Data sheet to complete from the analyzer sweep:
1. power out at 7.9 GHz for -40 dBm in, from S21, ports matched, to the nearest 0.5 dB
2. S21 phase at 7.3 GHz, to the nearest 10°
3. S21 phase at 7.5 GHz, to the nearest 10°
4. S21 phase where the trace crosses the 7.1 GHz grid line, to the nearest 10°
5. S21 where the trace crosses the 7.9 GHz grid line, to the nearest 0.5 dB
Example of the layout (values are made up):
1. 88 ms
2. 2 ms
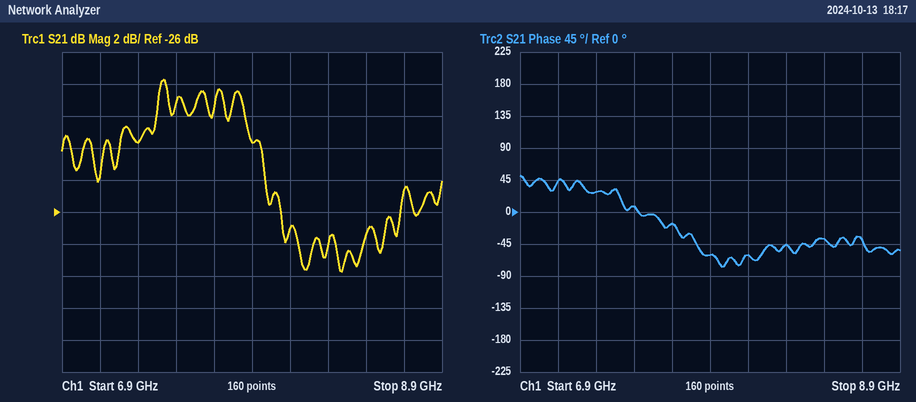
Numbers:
1. -61.5 dBm
2. 30°
3. 10°
4. 40°
5. -21.5 dB
